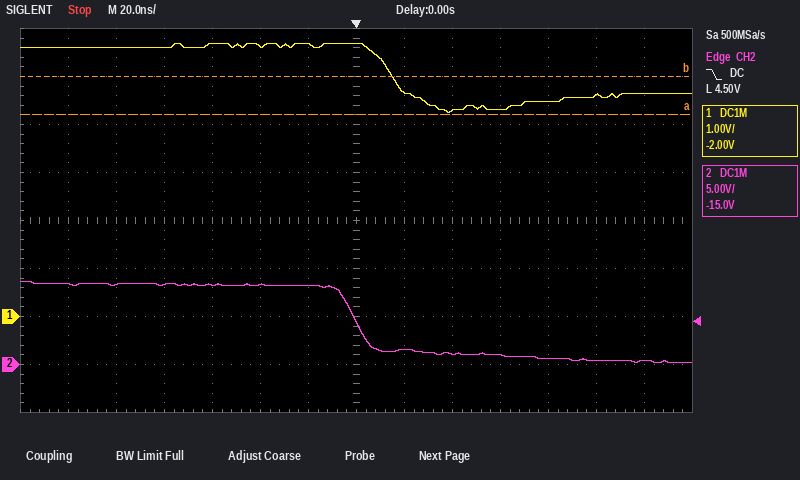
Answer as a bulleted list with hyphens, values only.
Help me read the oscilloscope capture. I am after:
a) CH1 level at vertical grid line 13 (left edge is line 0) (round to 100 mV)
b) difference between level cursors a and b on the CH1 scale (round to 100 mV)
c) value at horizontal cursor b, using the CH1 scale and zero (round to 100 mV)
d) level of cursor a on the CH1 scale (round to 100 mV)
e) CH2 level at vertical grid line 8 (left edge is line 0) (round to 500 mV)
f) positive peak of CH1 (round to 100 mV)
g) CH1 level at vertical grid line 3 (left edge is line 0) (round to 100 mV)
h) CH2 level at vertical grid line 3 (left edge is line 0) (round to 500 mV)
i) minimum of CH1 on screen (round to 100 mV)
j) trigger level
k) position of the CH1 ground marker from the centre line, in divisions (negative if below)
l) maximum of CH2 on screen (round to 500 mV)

- 4.6 V
- 800 mV
- 5.0 V
- 4.2 V
- 1.5 V
- 5.7 V
- 5.6 V
- 8.5 V
- 4.2 V
- 4.50 V
- -2.0 div
- 8.5 V
